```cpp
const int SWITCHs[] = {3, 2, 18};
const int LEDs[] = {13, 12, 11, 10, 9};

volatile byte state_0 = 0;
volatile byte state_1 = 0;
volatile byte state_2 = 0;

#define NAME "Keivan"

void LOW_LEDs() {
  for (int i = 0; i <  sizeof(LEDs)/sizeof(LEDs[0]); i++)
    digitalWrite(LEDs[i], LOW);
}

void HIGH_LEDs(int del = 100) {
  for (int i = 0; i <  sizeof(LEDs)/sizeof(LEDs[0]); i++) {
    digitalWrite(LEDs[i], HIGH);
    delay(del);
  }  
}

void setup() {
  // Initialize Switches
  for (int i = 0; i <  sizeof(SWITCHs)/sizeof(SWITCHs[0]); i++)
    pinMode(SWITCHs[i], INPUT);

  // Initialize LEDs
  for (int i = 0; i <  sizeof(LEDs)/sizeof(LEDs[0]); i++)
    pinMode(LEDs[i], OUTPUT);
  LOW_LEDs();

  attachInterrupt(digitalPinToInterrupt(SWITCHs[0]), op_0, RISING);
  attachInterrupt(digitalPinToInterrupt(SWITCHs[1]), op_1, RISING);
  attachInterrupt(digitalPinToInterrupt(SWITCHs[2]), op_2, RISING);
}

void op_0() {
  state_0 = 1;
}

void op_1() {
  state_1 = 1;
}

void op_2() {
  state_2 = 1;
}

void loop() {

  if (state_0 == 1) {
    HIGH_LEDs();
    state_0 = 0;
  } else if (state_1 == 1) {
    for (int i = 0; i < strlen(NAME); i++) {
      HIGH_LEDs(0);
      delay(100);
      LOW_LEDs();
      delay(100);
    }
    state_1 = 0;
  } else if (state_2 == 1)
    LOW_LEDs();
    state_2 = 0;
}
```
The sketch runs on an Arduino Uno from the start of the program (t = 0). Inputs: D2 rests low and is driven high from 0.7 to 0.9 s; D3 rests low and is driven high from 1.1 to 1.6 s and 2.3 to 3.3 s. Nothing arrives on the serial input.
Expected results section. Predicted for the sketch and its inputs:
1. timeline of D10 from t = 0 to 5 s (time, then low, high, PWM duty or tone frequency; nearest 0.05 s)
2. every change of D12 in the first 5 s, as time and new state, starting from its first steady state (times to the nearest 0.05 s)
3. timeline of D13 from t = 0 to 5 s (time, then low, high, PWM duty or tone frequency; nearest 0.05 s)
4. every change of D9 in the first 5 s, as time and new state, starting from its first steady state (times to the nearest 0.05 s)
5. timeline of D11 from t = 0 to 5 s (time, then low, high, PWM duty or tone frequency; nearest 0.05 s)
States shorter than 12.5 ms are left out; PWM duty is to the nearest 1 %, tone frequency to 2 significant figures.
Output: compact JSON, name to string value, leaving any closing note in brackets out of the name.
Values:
{"timeline of D10 from t = 0 to 5 s": "0 s low; 0.7 s high; 0.8 s low; 0.9 s high; 1 s low; 1.1 s high; 1.2 s low; 1.3 s high; 1.4 s low; 1.5 s high; 1.6 s low; 1.7 s high; 1.8 s low; 2.2 s high", "every change of D12 in the first 5 s, as time and new state, starting from its first steady state": "0 s low; 0.7 s high; 0.8 s low; 0.9 s high; 1 s low; 1.1 s high; 1.2 s low; 1.3 s high; 1.4 s low; 1.5 s high; 1.6 s low; 1.7 s high; 1.8 s low; 2 s high", "timeline of D13 from t = 0 to 5 s": "0 s low; 0.7 s high; 0.8 s low; 0.9 s high; 1 s low; 1.1 s high; 1.2 s low; 1.3 s high; 1.4 s low; 1.5 s high; 1.6 s low; 1.7 s high; 1.8 s low; 1.9 s high", "every change of D9 in the first 5 s, as time and new state, starting from its first steady state": "0 s low; 0.7 s high; 0.8 s low; 0.9 s high; 1 s low; 1.1 s high; 1.2 s low; 1.3 s high; 1.4 s low; 1.5 s high; 1.6 s low; 1.7 s high; 1.8 s low; 2.3 s high", "timeline of D11 from t = 0 to 5 s": "0 s low; 0.7 s high; 0.8 s low; 0.9 s high; 1 s low; 1.1 s high; 1.2 s low; 1.3 s high; 1.4 s low; 1.5 s high; 1.6 s low; 1.7 s high; 1.8 s low; 2.1 s high"}
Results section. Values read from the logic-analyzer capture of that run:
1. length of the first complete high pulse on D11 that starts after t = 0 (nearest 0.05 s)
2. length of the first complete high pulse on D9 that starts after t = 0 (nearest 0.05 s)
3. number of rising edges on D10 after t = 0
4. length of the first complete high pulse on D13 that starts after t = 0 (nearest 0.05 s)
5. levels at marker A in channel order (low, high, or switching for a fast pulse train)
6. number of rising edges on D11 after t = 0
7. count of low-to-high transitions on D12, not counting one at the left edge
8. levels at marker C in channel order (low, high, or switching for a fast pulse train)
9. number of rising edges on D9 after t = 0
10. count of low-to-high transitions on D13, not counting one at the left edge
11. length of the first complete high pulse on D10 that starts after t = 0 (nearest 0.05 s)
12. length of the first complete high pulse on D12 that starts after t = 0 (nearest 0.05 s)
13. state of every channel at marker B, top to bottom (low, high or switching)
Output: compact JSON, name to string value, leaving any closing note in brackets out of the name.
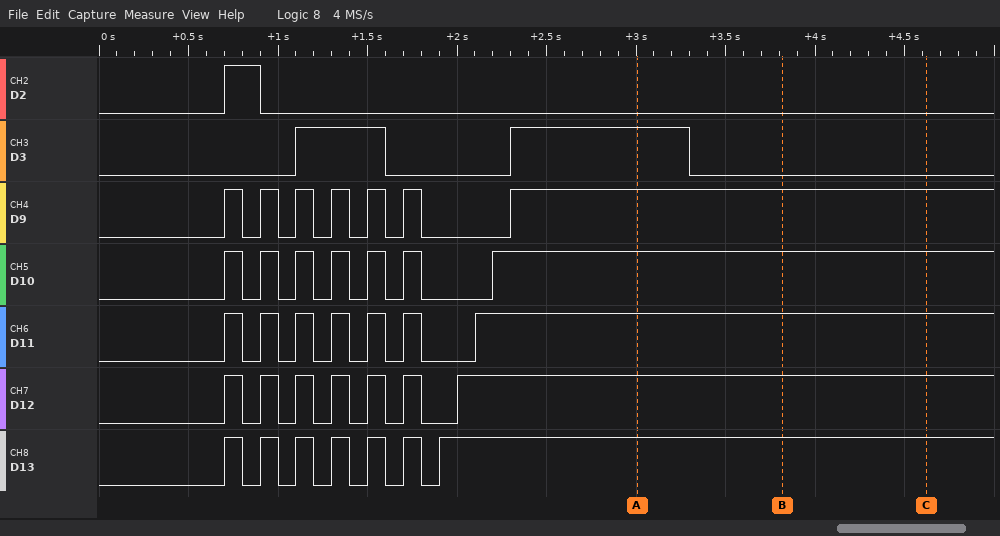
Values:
{"length of the first complete high pulse on D11 that starts after t = 0": "0.10 s", "length of the first complete high pulse on D9 that starts after t = 0": "0.10 s", "number of rising edges on D10 after t = 0": "7", "length of the first complete high pulse on D13 that starts after t = 0": "0.10 s", "levels at marker A in channel order": "D2 low, D3 high, D9 high, D10 high, D11 high, D12 high, D13 high", "number of rising edges on D11 after t = 0": "7", "count of low-to-high transitions on D12, not counting one at the left edge": "7", "levels at marker C in channel order": "D2 low, D3 low, D9 high, D10 high, D11 high, D12 high, D13 high", "number of rising edges on D9 after t = 0": "7", "count of low-to-high transitions on D13, not counting one at the left edge": "7", "length of the first complete high pulse on D10 that starts after t = 0": "0.10 s", "length of the first complete high pulse on D12 that starts after t = 0": "0.10 s", "state of every channel at marker B, top to bottom": "D2 low, D3 low, D9 high, D10 high, D11 high, D12 high, D13 high"}
